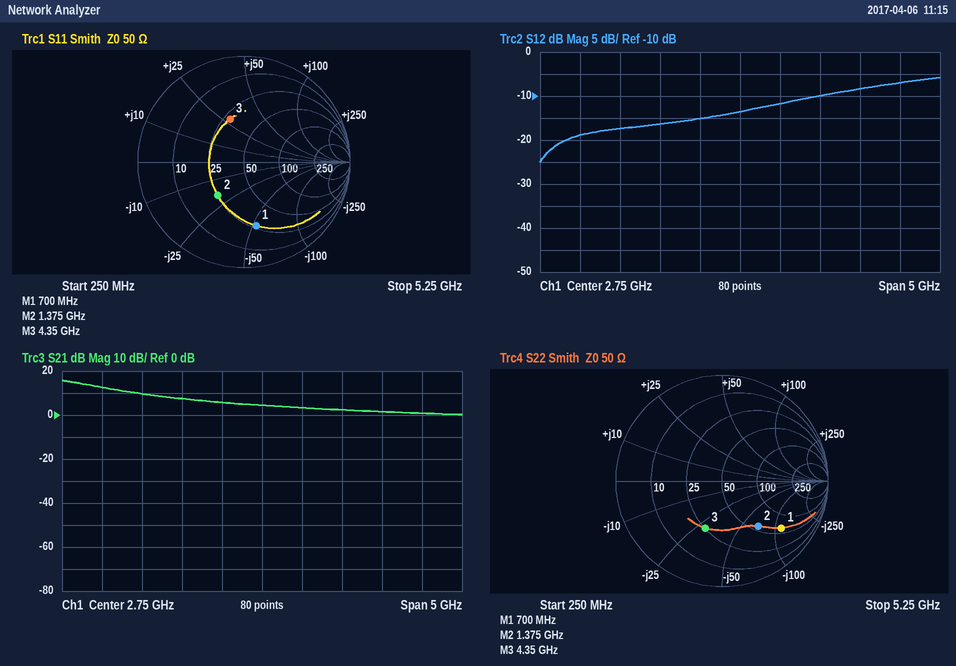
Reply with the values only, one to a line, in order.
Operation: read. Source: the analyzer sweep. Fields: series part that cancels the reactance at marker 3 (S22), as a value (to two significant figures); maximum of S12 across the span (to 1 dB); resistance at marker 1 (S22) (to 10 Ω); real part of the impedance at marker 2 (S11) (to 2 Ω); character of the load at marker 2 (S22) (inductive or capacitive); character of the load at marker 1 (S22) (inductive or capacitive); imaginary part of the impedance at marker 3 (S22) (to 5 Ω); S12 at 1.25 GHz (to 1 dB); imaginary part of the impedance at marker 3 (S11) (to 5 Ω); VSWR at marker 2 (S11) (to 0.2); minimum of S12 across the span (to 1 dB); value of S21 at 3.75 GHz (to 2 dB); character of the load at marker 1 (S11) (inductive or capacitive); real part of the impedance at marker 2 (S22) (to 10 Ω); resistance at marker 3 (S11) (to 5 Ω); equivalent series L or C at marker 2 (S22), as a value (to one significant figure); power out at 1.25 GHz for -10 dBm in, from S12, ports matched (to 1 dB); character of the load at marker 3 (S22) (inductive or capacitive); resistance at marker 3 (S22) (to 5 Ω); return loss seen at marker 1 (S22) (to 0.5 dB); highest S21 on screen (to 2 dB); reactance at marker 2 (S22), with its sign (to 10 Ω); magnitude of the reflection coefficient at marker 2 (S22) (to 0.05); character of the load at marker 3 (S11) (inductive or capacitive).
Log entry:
1.1 nH
-6 dB
60 Ω
26 Ω
capacitive
capacitive
-30 Ω
-17 dB
+30 Ω
2.4
-25 dB
2 dB
capacitive
60 Ω
30 Ω
2 pF
-27 dBm
capacitive
25 Ω
3.0 dB
16 dB
-70 Ω
0.55
inductive
